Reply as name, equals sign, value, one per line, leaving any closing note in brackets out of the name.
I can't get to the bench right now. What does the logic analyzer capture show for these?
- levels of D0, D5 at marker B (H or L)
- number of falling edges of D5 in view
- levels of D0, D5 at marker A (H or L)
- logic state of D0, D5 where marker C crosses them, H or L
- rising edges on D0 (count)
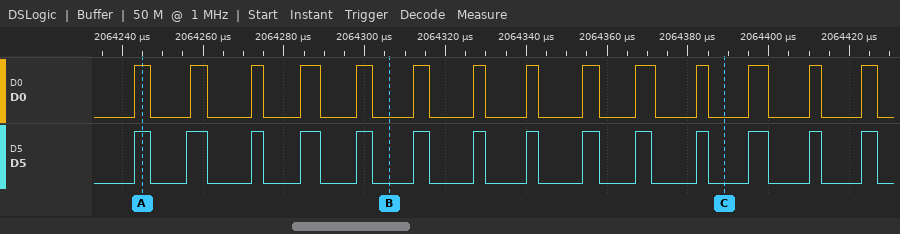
levels of D0, D5 at marker B = D0=L, D5=L
number of falling edges of D5 in view = 14
levels of D0, D5 at marker A = D0=H, D5=H
logic state of D0, D5 where marker C crosses them, H or L = D0=L, D5=L
rising edges on D0 = 14
